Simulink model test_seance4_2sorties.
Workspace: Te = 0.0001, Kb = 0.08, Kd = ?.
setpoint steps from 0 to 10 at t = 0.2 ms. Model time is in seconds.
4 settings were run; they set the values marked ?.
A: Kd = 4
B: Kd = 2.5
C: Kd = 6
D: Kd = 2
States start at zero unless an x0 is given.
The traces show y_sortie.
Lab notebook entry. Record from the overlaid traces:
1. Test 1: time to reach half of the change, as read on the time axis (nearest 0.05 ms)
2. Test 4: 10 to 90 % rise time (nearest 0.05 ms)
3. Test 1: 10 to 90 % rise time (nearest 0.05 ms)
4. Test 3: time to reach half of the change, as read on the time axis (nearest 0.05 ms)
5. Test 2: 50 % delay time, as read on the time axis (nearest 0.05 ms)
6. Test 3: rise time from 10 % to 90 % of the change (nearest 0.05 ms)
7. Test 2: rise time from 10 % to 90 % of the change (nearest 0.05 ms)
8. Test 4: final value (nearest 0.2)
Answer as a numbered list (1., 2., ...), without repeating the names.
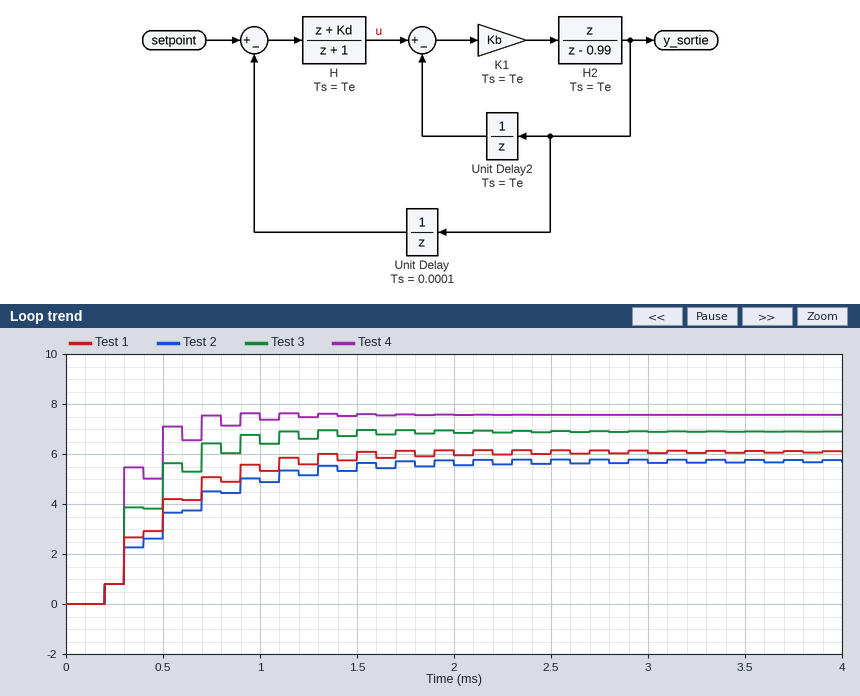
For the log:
1. 0.50 ms
2. 0.30 ms
3. 0.70 ms
4. 0.30 ms
5. 0.50 ms
6. 0.50 ms
7. 0.90 ms
8. 7.6
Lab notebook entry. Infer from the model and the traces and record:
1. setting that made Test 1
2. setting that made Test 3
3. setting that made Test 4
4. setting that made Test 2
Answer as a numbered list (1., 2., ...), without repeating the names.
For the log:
1. B
2. A
3. C
4. D
